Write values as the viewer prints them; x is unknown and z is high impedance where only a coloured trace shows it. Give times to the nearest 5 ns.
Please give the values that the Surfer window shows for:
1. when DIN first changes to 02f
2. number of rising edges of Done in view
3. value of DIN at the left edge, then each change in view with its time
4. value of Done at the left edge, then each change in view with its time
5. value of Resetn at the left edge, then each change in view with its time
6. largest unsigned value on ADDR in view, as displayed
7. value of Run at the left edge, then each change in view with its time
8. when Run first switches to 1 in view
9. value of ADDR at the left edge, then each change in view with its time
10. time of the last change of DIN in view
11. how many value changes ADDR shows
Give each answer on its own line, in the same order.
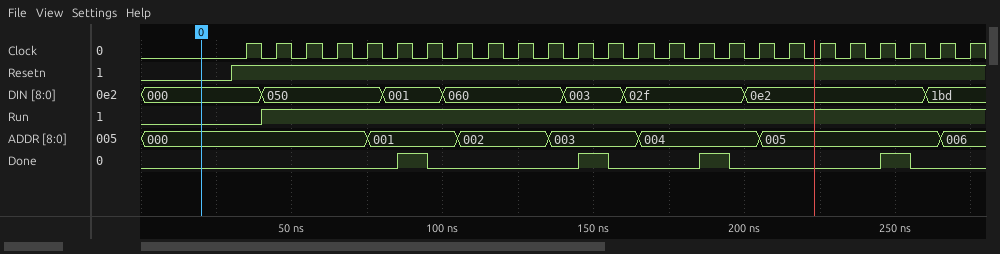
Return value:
160 ns
4
000, 050 at 40 ns, 001 at 80 ns, 060 at 100 ns, 003 at 140 ns, 02f at 160 ns, 0e2 at 200 ns, 1bd at 260 ns
0, 1 at 85 ns, 0 at 95 ns, 1 at 145 ns, 0 at 155 ns, 1 at 185 ns, 0 at 195 ns, 1 at 245 ns, 0 at 255 ns
0, 1 at 30 ns
006
0, 1 at 40 ns
40 ns
000, 001 at 75 ns, 002 at 105 ns, 003 at 135 ns, 004 at 165 ns, 005 at 205 ns, 006 at 265 ns
260 ns
6
